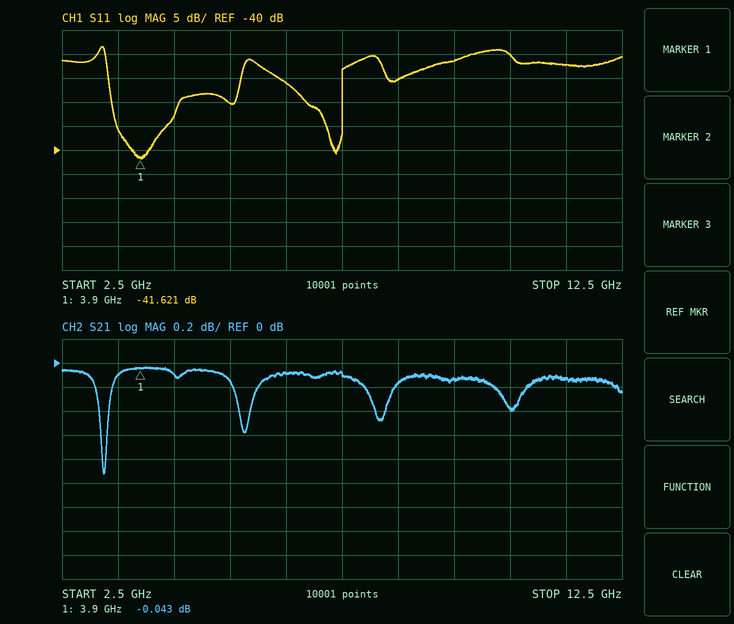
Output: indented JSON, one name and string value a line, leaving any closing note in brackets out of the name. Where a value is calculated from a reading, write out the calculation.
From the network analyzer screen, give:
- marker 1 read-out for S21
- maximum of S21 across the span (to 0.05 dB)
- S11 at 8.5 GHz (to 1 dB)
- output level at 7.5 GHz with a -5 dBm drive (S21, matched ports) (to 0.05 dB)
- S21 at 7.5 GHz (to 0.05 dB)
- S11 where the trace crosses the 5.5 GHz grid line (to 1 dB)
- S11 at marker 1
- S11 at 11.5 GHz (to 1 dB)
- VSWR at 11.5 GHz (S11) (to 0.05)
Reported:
{
  "marker 1 read-out for S21": "-0.043 dB",
  "maximum of S21 across the span": "-0.05 dB",
  "S11 at 8.5 GHz": "-25 dB",
  "output level at 7.5 GHz with a -5 dBm drive (S21, matched ports)": "-5 dBm + (-0.10 dB) = -5.10 dBm",
  "S21 at 7.5 GHz": "-0.10 dB",
  "S11 where the trace crosses the 5.5 GHz grid line": "-30 dB",
  "S11 at marker 1": "-41.621 dB",
  "S11 at 11.5 GHz": "-22 dB",
  "VSWR at 11.5 GHz (S11)": "|Γ| = 10^(-22/20) = 0.0794; VSWR = (1 + 0.0794)/(1 − 0.0794) ≈ 1.17, so 1.15 to the nearest 0.05"
}
